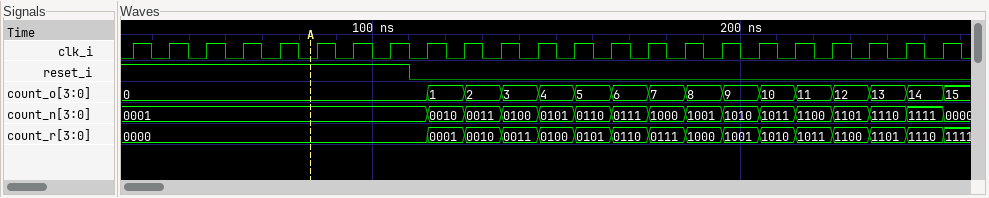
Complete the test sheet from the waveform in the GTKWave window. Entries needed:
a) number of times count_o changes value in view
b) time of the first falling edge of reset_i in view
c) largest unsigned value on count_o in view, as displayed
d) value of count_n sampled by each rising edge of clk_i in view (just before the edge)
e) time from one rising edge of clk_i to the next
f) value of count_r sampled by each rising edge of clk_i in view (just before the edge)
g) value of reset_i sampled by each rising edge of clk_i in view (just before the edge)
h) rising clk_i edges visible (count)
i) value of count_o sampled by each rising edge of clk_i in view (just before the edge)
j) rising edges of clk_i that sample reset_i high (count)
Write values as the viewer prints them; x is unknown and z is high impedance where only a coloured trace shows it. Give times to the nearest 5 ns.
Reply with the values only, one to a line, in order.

15
110 ns
15
0001, 0001, 0001, 0001, 0001, 0001, 0001, 0001, 0001, 0010, 0011, 0100, 0101, 0110, 0111, 1000, 1001, 1010, 1011, 1100, 1101, 1110, 1111
10 ns
0000, 0000, 0000, 0000, 0000, 0000, 0000, 0000, 0000, 0001, 0010, 0011, 0100, 0101, 0110, 0111, 1000, 1001, 1010, 1011, 1100, 1101, 1110
1 1 1 1 1 1 1 1 0 0 0 0 0 0 0 0 0 0 0 0 0 0 0
23
0, 0, 0, 0, 0, 0, 0, 0, 0, 1, 2, 3, 4, 5, 6, 7, 8, 9, 10, 11, 12, 13, 14
8
